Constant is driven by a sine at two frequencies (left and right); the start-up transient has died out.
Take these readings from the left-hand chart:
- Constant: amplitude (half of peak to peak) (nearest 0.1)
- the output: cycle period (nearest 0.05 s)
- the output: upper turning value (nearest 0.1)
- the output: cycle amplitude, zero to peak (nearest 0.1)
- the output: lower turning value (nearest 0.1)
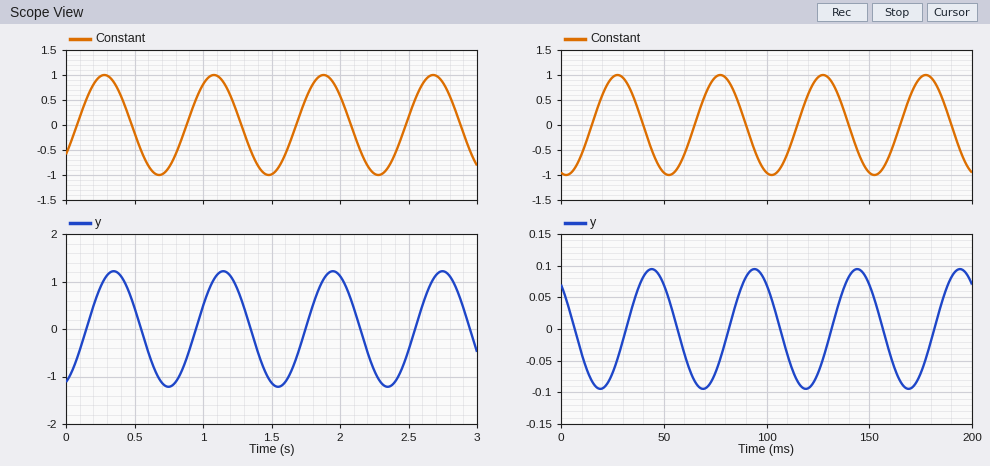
1.0
0.80 s
1.2
1.2
-1.2
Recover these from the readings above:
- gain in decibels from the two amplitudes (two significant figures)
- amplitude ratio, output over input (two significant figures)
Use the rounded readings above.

1.6 dB
1.2
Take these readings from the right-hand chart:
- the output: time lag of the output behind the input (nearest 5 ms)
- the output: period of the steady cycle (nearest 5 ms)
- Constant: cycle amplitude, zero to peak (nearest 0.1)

15 ms
50 ms
1.0
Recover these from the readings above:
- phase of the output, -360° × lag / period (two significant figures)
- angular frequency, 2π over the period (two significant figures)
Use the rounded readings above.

-110°
0.13 rad/ms
